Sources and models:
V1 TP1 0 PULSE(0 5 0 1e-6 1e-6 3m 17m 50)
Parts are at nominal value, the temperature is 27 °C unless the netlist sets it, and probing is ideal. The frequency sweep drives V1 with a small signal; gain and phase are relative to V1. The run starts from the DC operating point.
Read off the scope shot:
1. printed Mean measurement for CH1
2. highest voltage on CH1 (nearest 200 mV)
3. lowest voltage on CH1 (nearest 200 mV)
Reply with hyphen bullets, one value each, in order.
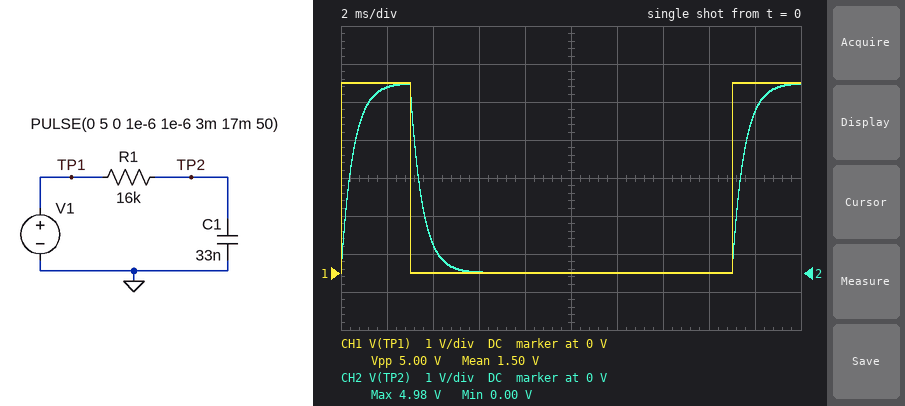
- 1.50 V
- 5.0 V
- 0 V
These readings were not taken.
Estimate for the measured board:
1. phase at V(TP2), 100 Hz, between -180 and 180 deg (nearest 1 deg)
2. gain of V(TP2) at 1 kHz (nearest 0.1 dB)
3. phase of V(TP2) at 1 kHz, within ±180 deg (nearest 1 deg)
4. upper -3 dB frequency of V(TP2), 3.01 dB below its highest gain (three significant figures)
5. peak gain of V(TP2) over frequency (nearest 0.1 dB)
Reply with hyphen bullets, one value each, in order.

- -18 deg
- -10.8 dB
- -73 deg
- 301 Hz
- 0 dB
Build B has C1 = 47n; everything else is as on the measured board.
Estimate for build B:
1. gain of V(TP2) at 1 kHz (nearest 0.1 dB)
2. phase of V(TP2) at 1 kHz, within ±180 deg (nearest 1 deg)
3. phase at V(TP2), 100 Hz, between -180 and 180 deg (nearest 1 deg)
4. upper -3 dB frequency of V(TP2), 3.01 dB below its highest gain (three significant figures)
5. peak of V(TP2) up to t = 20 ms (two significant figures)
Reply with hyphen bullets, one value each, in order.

- -13.7 dB
- -78 deg
- -25 deg
- 212 Hz
- 4.9 V
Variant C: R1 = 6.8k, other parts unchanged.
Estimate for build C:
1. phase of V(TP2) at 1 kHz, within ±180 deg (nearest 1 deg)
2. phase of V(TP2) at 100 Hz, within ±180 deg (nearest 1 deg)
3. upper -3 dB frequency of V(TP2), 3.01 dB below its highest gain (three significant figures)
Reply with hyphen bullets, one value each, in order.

- -55 deg
- -8 deg
- 709 Hz
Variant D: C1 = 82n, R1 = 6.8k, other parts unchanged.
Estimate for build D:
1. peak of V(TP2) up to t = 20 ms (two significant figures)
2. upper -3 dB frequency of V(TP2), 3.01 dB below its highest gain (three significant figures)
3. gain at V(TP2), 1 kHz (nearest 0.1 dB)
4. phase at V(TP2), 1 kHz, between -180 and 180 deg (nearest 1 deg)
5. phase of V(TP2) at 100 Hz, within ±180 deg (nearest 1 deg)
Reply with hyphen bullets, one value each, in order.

- 5.0 V
- 285 Hz
- -11.2 dB
- -74 deg
- -19 deg
